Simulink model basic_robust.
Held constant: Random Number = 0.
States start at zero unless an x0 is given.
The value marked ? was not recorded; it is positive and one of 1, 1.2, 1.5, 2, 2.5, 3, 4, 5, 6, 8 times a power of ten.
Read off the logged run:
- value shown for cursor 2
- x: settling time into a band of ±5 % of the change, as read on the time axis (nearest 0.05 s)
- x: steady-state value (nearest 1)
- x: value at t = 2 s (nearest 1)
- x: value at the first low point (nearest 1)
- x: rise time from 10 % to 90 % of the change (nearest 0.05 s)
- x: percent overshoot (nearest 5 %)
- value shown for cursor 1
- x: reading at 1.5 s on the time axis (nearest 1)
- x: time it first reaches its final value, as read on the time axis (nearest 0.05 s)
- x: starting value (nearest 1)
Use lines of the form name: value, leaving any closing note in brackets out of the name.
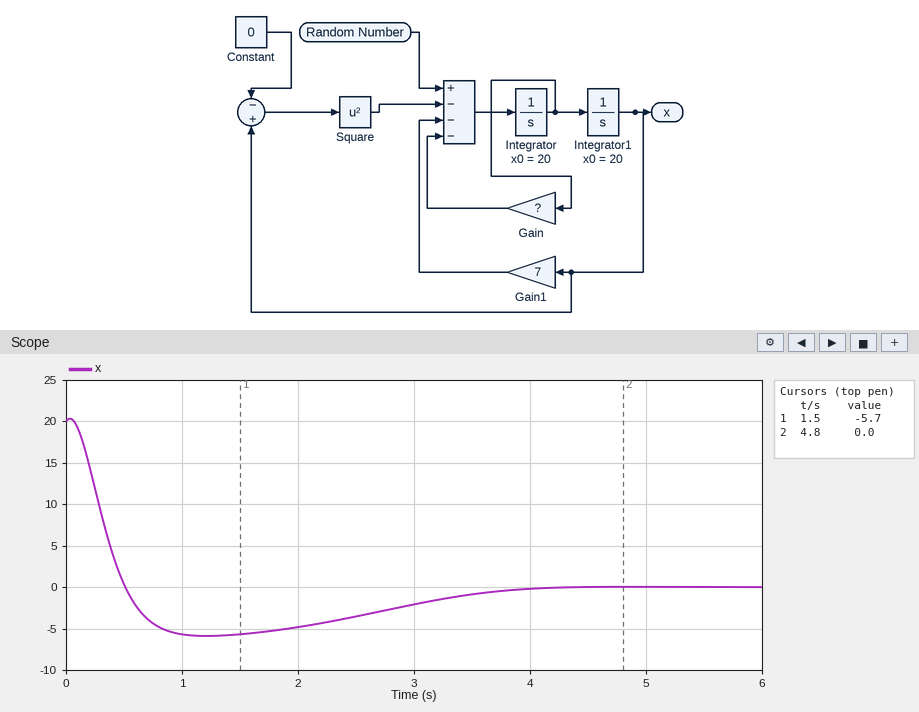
value shown for cursor 2: 0.0
x: settling time into a band of ±5 % of the change, as read on the time axis: 3.45 s
x: steady-state value: 0
x: value at t = 2 s: -5
x: value at the first low point: -6
x: rise time from 10 % to 90 % of the change: 0.30 s
x: percent overshoot: 30 %
value shown for cursor 1: -5.7
x: reading at 1.5 s on the time axis: -6
x: time it first reaches its final value, as read on the time axis: 0.50 s
x: starting value: 20
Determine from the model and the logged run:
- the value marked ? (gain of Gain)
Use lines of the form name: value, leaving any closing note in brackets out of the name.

the value marked ?: 4
